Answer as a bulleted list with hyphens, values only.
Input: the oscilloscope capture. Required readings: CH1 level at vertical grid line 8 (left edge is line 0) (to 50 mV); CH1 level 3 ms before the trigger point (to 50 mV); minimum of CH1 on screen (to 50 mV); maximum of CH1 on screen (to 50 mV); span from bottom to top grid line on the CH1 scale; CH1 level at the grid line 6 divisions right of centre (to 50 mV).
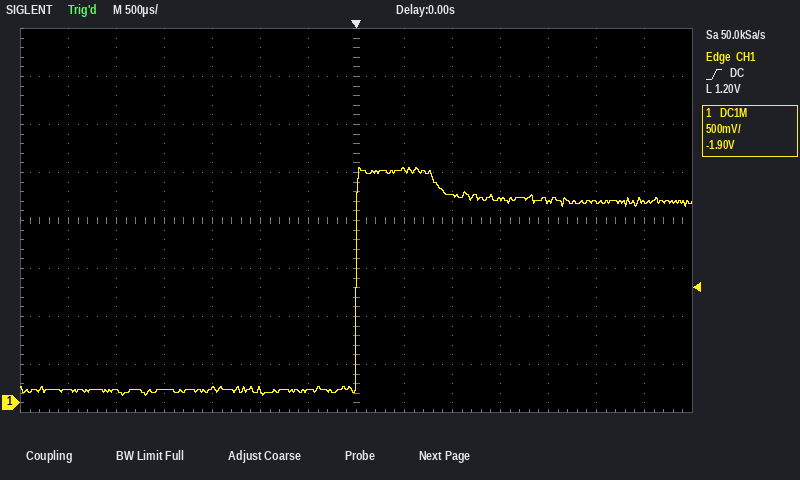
- 2.45 V
- 150 mV
- 100 mV
- 2.45 V
- 4 V
- 2.10 V
